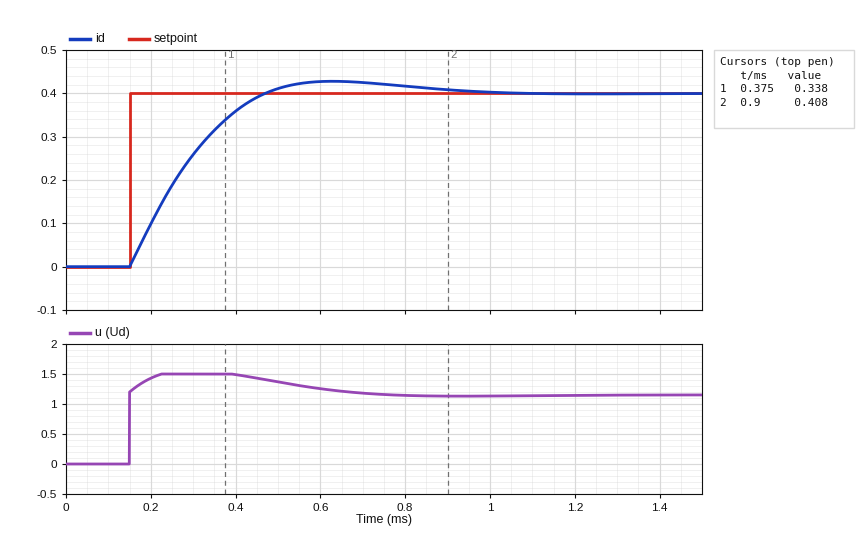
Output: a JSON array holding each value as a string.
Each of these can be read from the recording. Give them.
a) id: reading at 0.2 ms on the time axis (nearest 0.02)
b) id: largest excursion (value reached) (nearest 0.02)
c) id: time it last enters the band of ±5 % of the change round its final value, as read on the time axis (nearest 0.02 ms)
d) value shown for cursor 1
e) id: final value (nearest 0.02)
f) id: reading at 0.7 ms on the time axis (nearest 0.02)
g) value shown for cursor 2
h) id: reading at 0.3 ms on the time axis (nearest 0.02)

["0.10", "0.42", "0.76 ms", "0.338", "0.40", "0.42", "0.408", "0.26"]
